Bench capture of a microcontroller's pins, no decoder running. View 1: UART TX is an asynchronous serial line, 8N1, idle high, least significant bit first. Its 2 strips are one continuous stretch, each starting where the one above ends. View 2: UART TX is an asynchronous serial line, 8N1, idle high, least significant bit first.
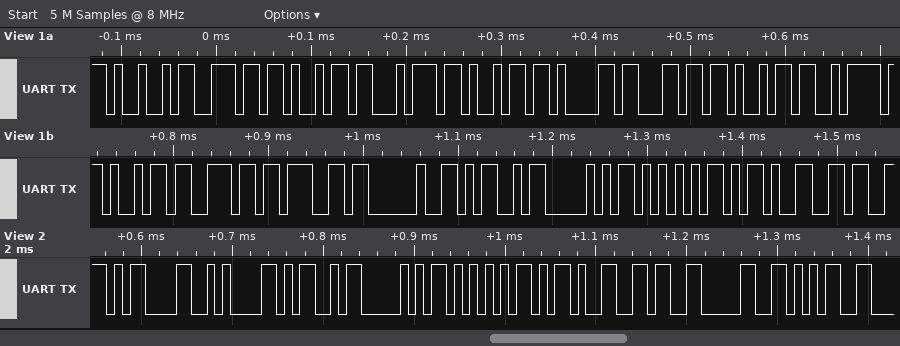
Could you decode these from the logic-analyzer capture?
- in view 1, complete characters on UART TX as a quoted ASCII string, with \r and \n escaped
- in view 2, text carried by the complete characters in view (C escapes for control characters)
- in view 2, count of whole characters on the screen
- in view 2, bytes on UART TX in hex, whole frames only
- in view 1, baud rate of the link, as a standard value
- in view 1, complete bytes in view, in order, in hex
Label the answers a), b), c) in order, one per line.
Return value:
a) "Initializing MPU-6"
b) "\r\nMPU-605"
c) 9
d) 0D 0A 4D 50 55 2D 36 30 35
e) 115200 baud
f) 49 6E 69 74 69 61 6C 69 7A 69 6E 67 20 4D 50 55 2D 36
